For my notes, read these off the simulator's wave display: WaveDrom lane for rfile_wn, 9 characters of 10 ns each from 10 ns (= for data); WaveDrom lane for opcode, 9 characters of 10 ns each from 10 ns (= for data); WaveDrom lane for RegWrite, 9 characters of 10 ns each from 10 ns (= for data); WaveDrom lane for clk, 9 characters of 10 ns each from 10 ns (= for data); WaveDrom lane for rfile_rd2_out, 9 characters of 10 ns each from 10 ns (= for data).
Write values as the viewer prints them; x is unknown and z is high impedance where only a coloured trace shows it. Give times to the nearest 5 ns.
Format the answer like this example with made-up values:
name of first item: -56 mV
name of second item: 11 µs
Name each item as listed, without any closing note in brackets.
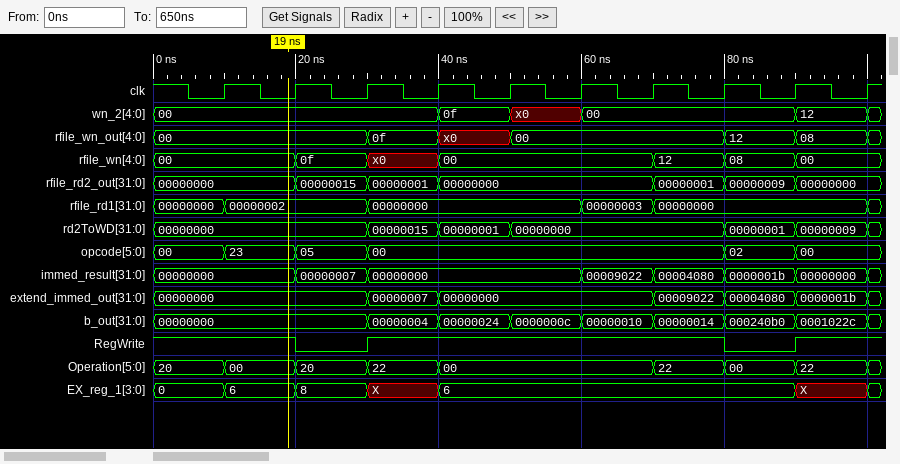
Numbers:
WaveDrom lane for rfile_wn, 9 characters of 10 ns each from 10 ns: {name: 'rfile_wn', wave: '====..===', data: '00 0f x0 00 12 08 00'}
WaveDrom lane for opcode, 9 characters of 10 ns each from 10 ns: {name: 'opcode', wave: '===....==', data: '23 05 00 02 00'}
WaveDrom lane for RegWrite, 9 characters of 10 ns each from 10 ns: {name: 'RegWrite', wave: '101....01'}
WaveDrom lane for clk, 9 characters of 10 ns each from 10 ns: {name: 'clk', wave: 'p........'}
WaveDrom lane for rfile_rd2_out, 9 characters of 10 ns each from 10 ns: {name: 'rfile_rd2_out', wave: '====..===', data: '00000000 00000015 00000001 00000000 00000001 00000009 00000000'}
